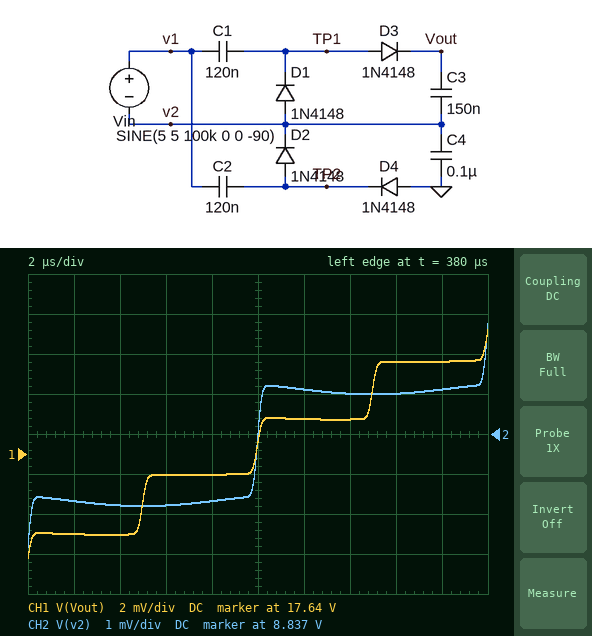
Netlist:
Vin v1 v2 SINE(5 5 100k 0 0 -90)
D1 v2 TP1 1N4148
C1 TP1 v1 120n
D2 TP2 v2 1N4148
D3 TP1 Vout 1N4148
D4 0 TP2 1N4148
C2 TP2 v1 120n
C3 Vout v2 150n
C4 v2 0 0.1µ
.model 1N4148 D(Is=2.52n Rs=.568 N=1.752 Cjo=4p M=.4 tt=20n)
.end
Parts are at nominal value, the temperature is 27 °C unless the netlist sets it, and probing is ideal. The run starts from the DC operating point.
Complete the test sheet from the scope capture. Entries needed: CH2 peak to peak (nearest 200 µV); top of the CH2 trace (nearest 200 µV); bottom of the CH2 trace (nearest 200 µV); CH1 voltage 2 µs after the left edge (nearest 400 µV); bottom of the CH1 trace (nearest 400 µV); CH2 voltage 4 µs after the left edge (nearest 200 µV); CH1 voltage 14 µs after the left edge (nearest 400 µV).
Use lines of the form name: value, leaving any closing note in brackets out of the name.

CH2 peak to peak: 5.6 mV
top of the CH2 trace: 8.8398 V
bottom of the CH2 trace: 8.8342 V
CH1 voltage 2 µs after the left edge: 17.6340 V
bottom of the CH1 trace: 17.6328 V
CH2 voltage 4 µs after the left edge: 8.8352 V
CH1 voltage 14 µs after the left edge: 17.6396 V
